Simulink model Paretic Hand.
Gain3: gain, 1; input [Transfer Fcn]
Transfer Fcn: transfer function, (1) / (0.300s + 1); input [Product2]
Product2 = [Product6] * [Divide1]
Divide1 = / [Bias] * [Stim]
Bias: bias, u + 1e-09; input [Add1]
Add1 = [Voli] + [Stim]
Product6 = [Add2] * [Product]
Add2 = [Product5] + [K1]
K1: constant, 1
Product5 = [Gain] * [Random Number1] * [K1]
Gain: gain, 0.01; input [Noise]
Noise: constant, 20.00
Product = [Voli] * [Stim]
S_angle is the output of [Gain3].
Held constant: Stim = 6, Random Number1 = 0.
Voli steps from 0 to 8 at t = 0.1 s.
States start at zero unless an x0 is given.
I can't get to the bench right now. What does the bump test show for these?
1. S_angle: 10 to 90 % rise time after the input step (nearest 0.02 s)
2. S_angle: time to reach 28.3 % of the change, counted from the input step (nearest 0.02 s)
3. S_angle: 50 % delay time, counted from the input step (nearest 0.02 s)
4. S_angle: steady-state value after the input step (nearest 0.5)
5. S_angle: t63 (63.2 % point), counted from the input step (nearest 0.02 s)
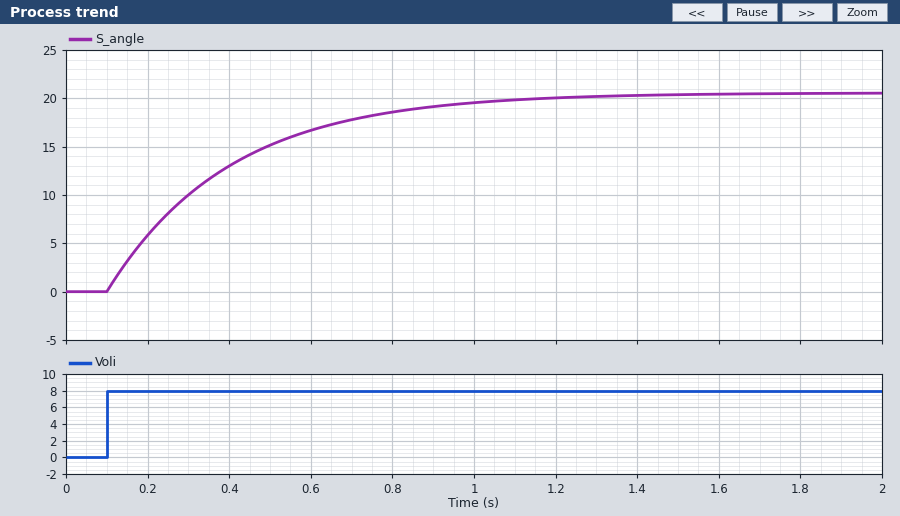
0.66 s
0.10 s
0.20 s
20.5
0.30 s
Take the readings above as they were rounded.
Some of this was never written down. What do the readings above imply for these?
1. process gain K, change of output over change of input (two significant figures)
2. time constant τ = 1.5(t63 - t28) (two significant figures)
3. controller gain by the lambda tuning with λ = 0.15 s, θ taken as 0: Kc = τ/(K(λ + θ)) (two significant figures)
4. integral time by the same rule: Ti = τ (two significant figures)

2.6
0.30 s
0.77
0.30 s
